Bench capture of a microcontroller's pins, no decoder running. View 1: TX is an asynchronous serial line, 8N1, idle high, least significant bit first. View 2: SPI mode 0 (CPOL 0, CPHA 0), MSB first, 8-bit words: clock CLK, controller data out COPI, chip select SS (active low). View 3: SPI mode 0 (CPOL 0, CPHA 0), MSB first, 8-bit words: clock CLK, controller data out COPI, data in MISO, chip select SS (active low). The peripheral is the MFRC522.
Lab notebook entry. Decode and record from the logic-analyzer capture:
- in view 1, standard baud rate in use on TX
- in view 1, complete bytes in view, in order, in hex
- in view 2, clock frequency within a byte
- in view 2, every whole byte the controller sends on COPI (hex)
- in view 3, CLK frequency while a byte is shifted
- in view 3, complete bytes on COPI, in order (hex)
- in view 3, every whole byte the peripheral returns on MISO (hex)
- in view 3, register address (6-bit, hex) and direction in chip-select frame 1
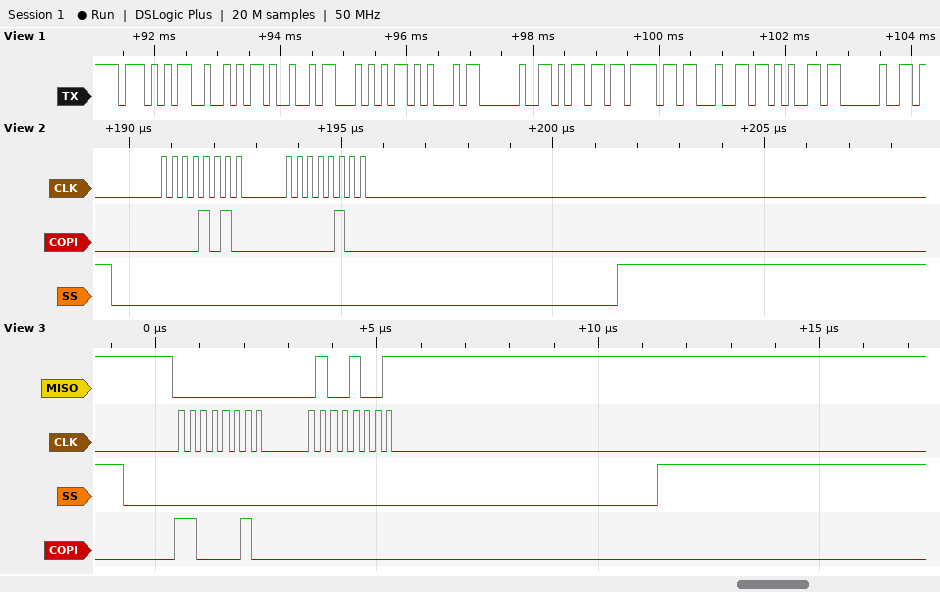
9600 baud
0x57 0x52 0x49 0x54 0x45 0x20 0x6D 0x6F 0x64 0x65 0x20
4 MHz
0A 04
4 MHz
0xC2 0x00
0x00 0x49
0x21 read
